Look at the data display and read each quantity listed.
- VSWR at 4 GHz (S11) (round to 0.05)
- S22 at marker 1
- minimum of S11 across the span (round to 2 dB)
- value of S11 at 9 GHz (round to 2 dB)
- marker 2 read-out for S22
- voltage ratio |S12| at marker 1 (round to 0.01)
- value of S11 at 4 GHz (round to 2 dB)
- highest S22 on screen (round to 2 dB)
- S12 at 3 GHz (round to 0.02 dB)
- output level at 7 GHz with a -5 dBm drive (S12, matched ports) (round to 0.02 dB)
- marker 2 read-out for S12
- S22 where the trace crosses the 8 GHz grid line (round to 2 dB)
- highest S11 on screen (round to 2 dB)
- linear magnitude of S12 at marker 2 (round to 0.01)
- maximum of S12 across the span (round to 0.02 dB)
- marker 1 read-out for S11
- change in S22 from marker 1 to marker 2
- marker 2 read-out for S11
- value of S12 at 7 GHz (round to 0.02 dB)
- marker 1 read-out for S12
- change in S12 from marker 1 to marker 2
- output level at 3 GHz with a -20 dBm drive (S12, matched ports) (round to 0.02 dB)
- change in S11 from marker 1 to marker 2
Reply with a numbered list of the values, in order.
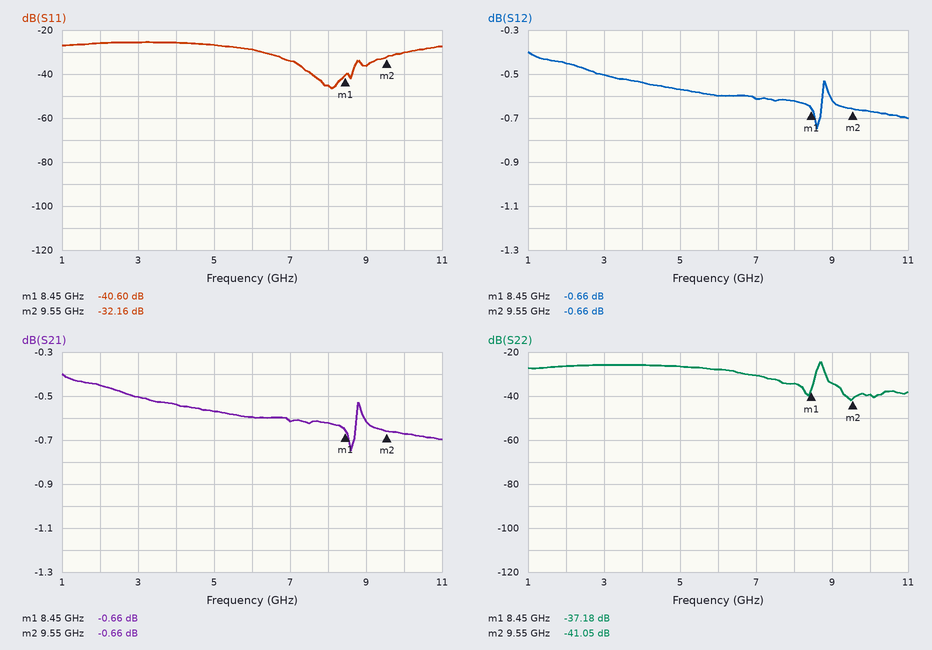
1. 1.10
2. -37.18 dB
3. -46 dB
4. -36 dB
5. -41.05 dB
6. 0.93
7. -26 dB
8. -24 dB
9. -0.50 dB
10. -5.62 dBm
11. -0.66 dB
12. -34 dB
13. -26 dB
14. 0.93
15. -0.40 dB
16. -40.60 dB
17. -3.87 dB
18. -32.16 dB
19. -0.62 dB
20. -0.66 dB
21. 0.00 dB
22. -20.50 dBm
23. 8.44 dB
